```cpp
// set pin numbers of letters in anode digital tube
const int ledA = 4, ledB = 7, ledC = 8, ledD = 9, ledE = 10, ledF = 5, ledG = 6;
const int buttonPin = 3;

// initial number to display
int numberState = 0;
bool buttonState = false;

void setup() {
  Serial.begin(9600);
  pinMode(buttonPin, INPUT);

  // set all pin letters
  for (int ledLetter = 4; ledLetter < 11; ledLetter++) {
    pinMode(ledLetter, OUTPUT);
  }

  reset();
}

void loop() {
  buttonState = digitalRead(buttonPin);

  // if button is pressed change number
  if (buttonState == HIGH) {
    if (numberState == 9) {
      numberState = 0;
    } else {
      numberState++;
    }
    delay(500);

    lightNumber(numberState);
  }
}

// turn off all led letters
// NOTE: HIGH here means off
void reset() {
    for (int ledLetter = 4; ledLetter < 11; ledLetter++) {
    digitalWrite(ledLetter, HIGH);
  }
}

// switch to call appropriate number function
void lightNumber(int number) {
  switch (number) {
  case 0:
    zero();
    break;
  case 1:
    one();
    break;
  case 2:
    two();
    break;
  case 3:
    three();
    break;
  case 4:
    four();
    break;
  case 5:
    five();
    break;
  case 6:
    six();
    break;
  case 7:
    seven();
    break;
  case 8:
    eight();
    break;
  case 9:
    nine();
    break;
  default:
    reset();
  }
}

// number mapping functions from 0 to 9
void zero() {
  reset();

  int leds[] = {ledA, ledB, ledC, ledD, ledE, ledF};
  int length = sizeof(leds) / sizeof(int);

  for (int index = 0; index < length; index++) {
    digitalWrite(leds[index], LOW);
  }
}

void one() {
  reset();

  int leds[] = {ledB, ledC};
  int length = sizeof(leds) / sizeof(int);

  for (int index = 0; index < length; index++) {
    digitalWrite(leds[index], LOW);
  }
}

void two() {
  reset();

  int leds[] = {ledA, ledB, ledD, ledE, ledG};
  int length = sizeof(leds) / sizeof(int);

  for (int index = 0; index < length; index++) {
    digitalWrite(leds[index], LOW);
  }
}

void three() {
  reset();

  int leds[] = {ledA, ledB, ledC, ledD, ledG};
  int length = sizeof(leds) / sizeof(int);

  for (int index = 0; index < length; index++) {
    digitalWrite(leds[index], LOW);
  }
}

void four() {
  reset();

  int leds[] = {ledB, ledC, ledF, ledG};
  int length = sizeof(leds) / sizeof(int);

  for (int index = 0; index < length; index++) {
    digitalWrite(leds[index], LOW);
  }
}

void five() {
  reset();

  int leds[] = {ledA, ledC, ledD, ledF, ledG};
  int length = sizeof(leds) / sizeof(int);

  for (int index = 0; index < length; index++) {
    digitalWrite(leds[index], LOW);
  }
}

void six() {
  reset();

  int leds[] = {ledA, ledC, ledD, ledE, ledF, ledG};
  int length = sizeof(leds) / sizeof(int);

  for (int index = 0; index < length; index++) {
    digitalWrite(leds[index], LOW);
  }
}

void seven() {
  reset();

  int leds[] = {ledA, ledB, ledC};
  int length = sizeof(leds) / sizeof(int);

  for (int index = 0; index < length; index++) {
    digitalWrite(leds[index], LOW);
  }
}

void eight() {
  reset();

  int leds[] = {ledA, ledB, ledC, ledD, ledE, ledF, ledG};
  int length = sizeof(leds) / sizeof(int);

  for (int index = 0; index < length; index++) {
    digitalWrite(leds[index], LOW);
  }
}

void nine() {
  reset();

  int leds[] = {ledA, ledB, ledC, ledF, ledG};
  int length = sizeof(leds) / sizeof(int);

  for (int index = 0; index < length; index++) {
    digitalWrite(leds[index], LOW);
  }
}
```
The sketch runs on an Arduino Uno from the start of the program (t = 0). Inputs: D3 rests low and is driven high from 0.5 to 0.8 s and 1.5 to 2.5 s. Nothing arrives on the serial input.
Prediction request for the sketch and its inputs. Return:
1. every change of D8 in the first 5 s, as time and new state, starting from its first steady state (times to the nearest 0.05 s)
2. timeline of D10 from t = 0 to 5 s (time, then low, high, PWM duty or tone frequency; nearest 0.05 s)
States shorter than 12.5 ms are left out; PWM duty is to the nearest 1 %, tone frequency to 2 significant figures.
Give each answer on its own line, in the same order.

0 s high; 1 s low; 2 s high; 2.5 s low
0 s high; 2 s low; 2.5 s high
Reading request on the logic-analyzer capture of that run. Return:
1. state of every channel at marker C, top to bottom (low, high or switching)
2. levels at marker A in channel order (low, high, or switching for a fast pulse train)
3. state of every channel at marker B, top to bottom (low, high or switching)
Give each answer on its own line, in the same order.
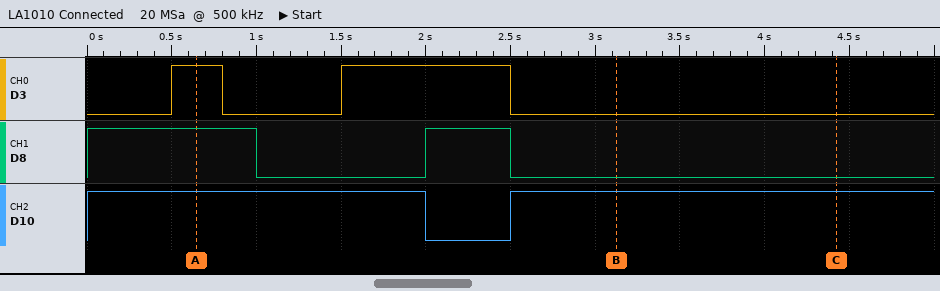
D3 low, D8 low, D10 high
D3 high, D8 high, D10 high
D3 low, D8 low, D10 high
